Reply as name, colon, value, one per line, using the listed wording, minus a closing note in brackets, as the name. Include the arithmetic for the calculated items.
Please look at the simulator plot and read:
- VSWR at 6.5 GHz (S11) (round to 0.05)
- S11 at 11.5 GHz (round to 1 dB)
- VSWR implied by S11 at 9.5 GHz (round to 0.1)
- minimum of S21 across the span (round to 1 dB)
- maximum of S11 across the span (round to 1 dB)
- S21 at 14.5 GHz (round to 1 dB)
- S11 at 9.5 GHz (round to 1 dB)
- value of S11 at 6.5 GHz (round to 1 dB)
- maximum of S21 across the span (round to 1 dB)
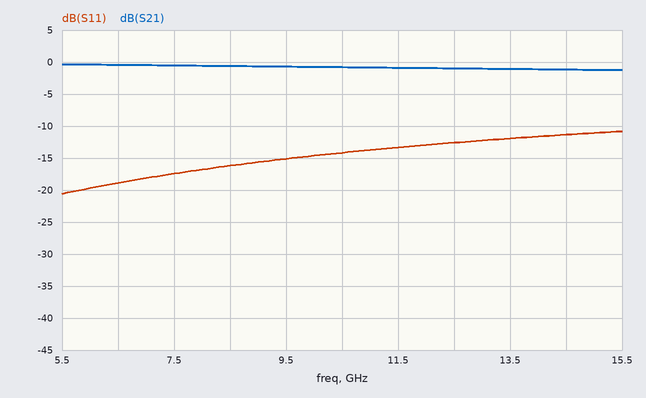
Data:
VSWR at 6.5 GHz (S11): |Γ| = 10^(-19/20) = 0.1122; VSWR = (1 + 0.1122)/(1 − 0.1122) ≈ 1.25
S11 at 11.5 GHz: -13 dB
VSWR implied by S11 at 9.5 GHz: |Γ| = 10^(-15/20) = 0.1778; VSWR = (1 + 0.1778)/(1 − 0.1778) ≈ 1.4
minimum of S21 across the span: -1 dB
maximum of S11 across the span: -11 dB
S21 at 14.5 GHz: -1 dB
S11 at 9.5 GHz: -15 dB
value of S11 at 6.5 GHz: -19 dB
maximum of S21 across the span: 0 dB
